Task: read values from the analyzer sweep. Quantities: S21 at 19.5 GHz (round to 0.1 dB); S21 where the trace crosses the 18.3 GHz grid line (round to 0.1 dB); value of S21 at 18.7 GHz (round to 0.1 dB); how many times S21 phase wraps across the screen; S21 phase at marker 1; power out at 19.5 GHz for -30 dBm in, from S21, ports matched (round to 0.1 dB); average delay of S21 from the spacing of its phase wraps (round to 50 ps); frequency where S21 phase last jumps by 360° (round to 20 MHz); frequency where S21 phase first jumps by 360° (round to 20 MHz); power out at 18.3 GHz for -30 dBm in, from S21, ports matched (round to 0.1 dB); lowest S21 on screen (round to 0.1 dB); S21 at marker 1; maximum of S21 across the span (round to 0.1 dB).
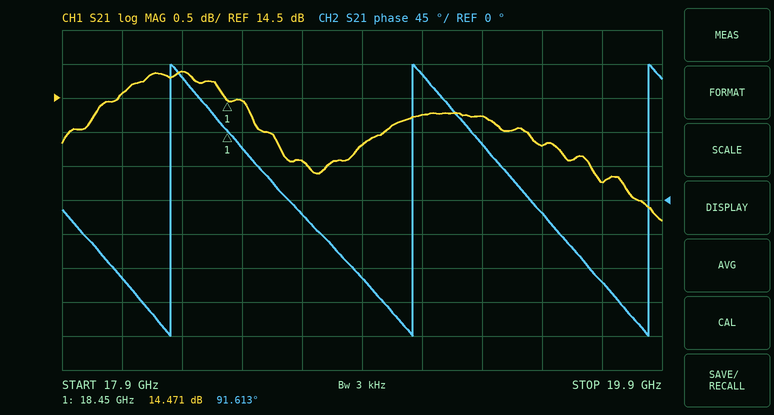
13.8 dB
14.9 dB
13.6 dB
3
91.613°
-16.2 dBm
1.25 ns
19.86 GHz
18.26 GHz
-15.1 dBm
12.7 dB
14.471 dB
14.9 dB
